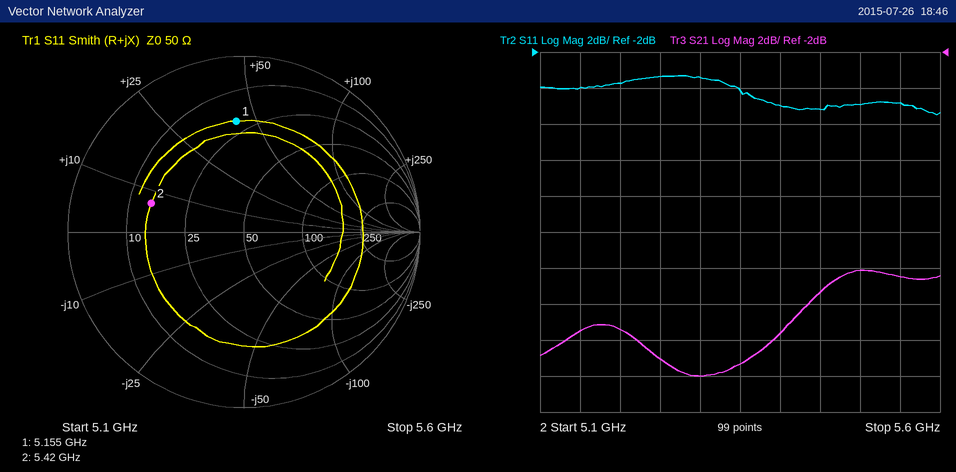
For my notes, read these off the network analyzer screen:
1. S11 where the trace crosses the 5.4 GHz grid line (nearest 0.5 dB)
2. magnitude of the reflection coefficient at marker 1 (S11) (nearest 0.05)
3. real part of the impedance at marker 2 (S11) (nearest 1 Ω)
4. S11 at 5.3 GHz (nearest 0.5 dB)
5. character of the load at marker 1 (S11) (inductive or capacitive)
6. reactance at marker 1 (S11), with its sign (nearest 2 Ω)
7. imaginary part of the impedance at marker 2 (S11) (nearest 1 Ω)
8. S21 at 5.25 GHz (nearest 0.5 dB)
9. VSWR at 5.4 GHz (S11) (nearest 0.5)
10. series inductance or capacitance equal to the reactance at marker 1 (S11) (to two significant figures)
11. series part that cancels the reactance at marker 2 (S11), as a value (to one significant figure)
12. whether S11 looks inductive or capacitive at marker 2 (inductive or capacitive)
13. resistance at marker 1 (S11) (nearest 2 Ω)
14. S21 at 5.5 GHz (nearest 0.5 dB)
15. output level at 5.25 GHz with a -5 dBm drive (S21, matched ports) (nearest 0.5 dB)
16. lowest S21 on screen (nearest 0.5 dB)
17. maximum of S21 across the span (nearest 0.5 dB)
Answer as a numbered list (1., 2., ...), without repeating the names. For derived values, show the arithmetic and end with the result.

1. -5.0 dB
2. 0.65
3. 15 Ω
4. -3.5 dB
5. inductive
6. +42 Ω
7. +7 Ω
8. -19.0 dB
9. |Γ| = 10^(-5/20) = 0.5623; VSWR = (1 + 0.5623)/(1 − 0.5623) ≈ 3.57, so 3.5 to the nearest 0.5
10. L = 42 Ω/(2π × 5.155 GHz) ≈ 1.3 nH
11. C = 1/(2π × 5.42 GHz × 7 Ω) ≈ 4 pF
12. inductive
13. 20 Ω
14. -14.0 dB
15. -5 dBm + (-19.0 dB) = -24.0 dBm
16. -20.0 dB
17. -14.0 dB
